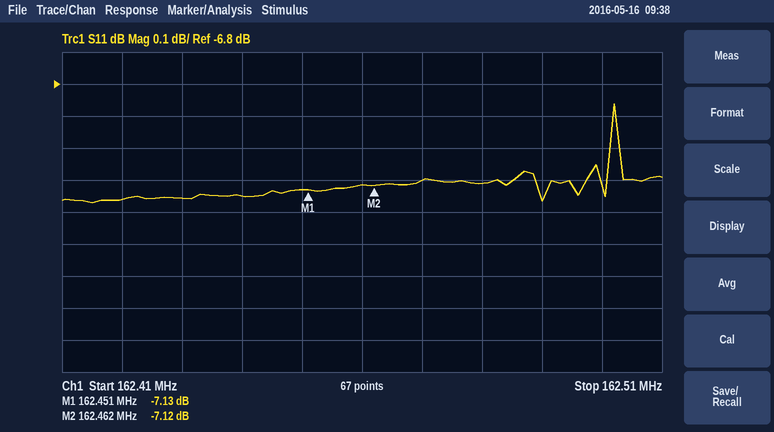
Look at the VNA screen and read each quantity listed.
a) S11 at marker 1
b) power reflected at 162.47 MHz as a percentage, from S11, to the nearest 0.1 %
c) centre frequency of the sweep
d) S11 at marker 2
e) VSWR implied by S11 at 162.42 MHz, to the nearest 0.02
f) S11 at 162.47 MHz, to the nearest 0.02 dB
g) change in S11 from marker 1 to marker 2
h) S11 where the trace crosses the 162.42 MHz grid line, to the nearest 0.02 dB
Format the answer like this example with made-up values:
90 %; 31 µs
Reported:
-7.13 dB; 19.5 %; 162.46 MHz; -7.12 dB; 2.56; -7.10 dB; 0.01 dB; -7.16 dB
